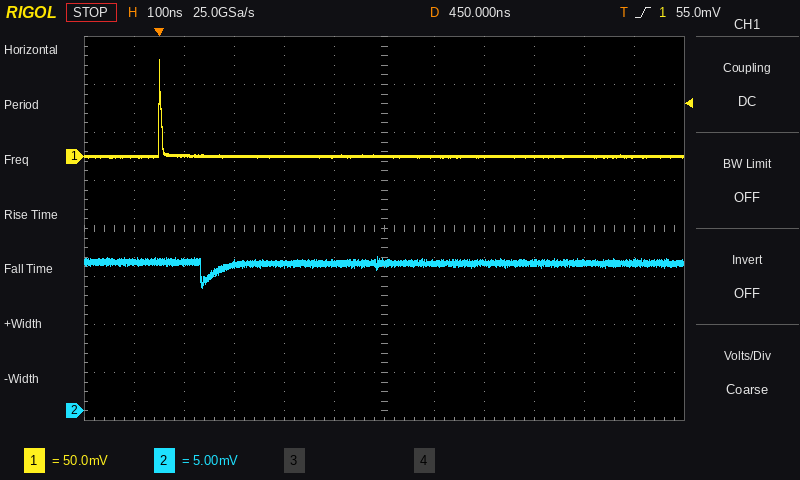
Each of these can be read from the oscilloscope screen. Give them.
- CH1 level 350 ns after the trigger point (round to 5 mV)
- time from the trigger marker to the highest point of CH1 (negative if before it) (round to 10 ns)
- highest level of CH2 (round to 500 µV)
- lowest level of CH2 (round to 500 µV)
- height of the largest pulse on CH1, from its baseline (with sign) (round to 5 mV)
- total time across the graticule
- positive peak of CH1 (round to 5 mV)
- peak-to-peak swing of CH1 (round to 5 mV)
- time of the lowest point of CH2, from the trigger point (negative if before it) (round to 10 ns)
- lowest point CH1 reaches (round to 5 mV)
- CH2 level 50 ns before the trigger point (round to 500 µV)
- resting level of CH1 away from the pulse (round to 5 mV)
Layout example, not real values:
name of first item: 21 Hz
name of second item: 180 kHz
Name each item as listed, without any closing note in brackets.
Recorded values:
CH1 level 350 ns after the trigger point: 0 mV
time from the trigger marker to the highest point of CH1 (negative if before it): 0 ns
highest level of CH2: 16.0 mV
lowest level of CH2: 13.0 mV
height of the largest pulse on CH1, from its baseline (with sign): +100 mV
total time across the graticule: 1.2 µs
positive peak of CH1: 100 mV
peak-to-peak swing of CH1: 100 mV
time of the lowest point of CH2, from the trigger point (negative if before it): +90 ns
lowest point CH1 reaches: 0 mV
CH2 level 50 ns before the trigger point: 15.5 mV
resting level of CH1 away from the pulse: 0 mV
